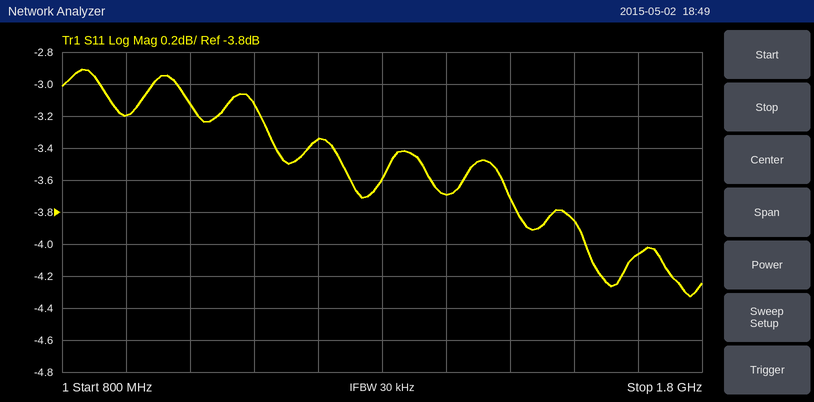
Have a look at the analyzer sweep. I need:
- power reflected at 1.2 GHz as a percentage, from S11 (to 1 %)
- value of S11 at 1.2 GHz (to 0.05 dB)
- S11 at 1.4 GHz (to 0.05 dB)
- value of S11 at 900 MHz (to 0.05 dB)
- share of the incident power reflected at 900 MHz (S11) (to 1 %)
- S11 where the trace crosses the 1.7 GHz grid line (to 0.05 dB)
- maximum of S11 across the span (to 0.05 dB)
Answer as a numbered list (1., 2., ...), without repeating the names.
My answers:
1. 46 %
2. -3.35 dB
3. -3.70 dB
4. -3.20 dB
5. 48 %
6. -4.05 dB
7. -2.90 dB
